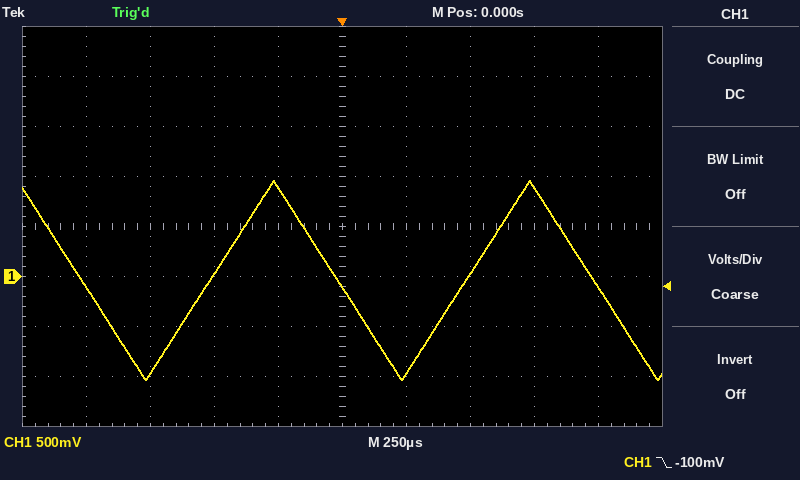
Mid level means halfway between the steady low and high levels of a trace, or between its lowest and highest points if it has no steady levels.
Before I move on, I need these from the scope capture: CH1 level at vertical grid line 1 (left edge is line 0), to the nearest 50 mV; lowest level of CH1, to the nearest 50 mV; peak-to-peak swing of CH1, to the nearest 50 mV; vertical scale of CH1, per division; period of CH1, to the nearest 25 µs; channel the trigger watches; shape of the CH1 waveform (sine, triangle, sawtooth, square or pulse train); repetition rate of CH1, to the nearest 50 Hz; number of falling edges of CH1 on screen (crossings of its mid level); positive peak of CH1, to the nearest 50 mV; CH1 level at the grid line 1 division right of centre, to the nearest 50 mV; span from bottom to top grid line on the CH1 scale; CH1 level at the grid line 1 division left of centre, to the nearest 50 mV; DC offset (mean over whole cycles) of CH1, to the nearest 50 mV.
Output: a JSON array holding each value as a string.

["-100 mV", "-1.05 V", "2.00 V", "500 mV", "1.000 ms", "CH1", "triangle", "1.00 kHz", "3", "950 mV", "-950 mV", "4 V", "900 mV", "-50 mV"]
